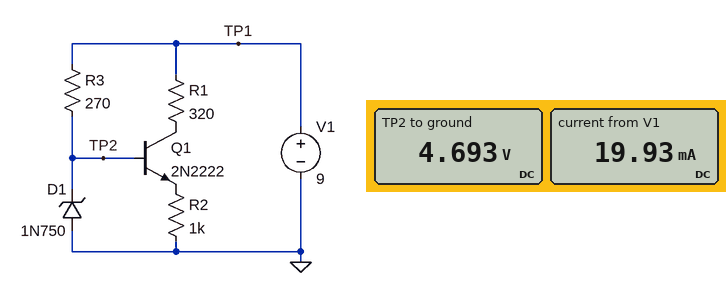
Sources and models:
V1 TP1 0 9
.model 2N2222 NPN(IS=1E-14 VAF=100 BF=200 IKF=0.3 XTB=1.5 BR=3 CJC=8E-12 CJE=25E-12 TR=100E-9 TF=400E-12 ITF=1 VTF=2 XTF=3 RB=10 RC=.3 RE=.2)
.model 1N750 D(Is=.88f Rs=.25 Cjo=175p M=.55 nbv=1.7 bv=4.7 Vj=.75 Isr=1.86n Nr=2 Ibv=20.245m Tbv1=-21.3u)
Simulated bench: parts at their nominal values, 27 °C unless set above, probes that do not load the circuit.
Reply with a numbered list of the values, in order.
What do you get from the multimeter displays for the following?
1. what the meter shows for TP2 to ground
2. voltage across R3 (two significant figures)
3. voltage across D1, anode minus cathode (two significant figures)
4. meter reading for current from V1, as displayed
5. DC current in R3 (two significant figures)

1. 4.693 V
2. 4.3 V
3. -4.7 V
4. 19.93 mA
5. 16 mA
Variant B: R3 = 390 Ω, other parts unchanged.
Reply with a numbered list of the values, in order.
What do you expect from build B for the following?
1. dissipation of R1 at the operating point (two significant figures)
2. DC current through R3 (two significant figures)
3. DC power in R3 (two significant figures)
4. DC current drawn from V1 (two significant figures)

1. 5.0 mW
2. 11 mA
3. 48 mW
4. 15 mA
